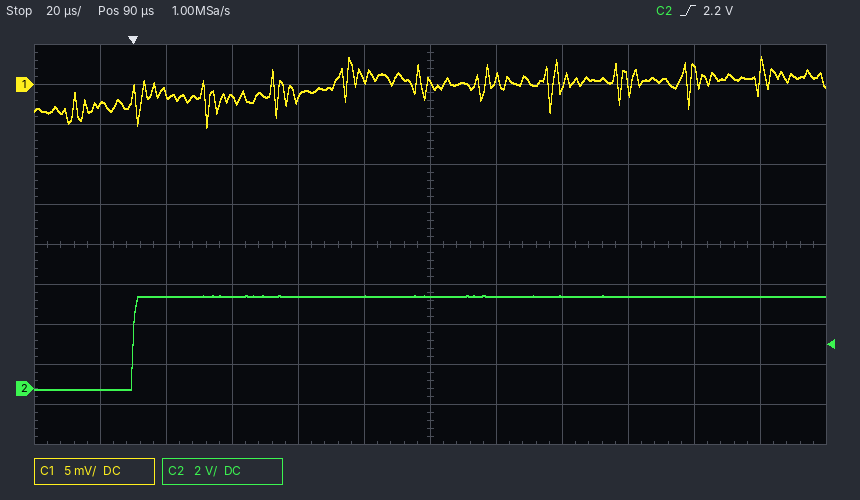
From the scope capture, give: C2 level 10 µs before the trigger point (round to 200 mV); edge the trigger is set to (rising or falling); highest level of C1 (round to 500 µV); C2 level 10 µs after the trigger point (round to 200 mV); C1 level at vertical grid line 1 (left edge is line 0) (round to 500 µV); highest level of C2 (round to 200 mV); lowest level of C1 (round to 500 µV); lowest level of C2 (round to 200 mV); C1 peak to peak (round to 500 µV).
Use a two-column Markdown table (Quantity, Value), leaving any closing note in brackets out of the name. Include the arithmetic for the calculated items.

| Quantity | Value |
|---|---|
| C2 level 10 µs before the trigger point | 0.0 V |
| edge the trigger is set to | rising |
| highest level of C1 | 3.5 mV |
| C2 level 10 µs after the trigger point | 4.6 V |
| C1 level at vertical grid line 1 (left edge is line 0) | -2.5 mV |
| highest level of C2 | 4.6 V |
| lowest level of C1 | -5.5 mV |
| lowest level of C2 | 0.0 V |
| C1 peak to peak | 3.5 mV − (-5.5 mV) = 9.0 mV |
